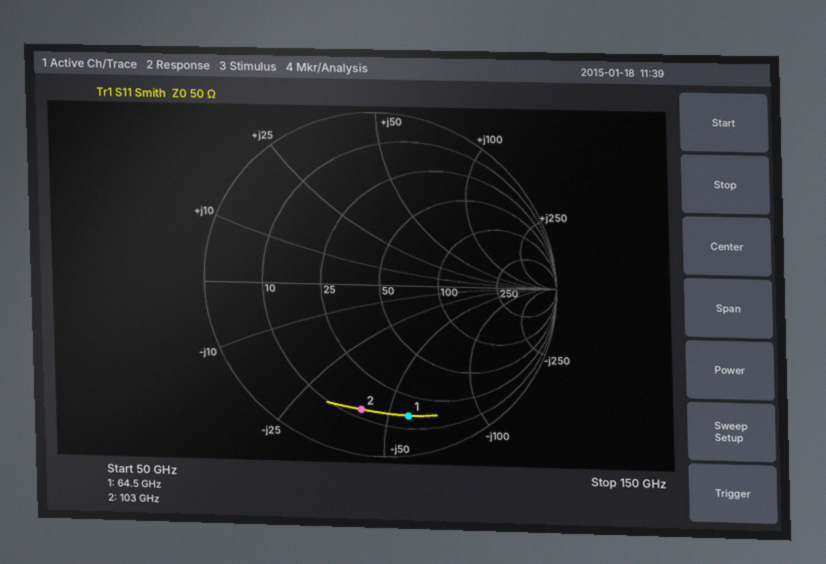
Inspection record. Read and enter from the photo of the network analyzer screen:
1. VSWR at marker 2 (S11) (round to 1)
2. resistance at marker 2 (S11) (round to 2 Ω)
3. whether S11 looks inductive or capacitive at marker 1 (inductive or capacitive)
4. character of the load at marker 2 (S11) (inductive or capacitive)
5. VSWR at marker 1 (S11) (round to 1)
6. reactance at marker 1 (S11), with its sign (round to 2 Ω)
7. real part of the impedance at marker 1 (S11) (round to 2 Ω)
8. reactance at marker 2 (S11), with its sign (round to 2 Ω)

7
12 Ω
capacitive
capacitive
8
-58 Ω
16 Ω
-40 Ω
